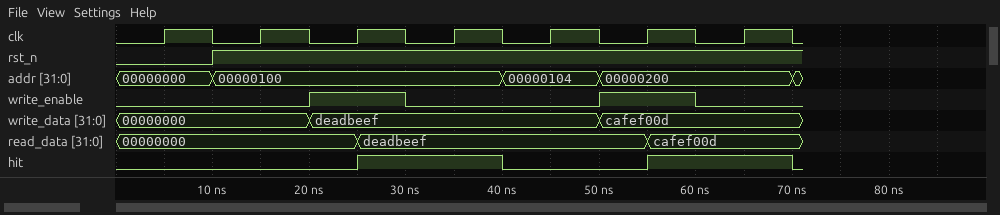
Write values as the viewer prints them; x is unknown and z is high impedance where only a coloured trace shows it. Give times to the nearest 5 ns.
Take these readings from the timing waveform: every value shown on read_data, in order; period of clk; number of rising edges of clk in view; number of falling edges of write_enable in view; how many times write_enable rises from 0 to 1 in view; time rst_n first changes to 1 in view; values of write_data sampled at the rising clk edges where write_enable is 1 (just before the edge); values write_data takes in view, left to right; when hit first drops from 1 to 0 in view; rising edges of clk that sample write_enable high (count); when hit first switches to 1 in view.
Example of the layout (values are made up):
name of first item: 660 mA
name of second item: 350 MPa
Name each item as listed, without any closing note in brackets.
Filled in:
every value shown on read_data, in order: 00000000, deadbeef, cafef00d
period of clk: 10 ns
number of rising edges of clk in view: 7
number of falling edges of write_enable in view: 2
how many times write_enable rises from 0 to 1 in view: 2
time rst_n first changes to 1 in view: 10 ns
values of write_data sampled at the rising clk edges where write_enable is 1: deadbeef, cafef00d
values write_data takes in view, left to right: 00000000, deadbeef, cafef00d
when hit first drops from 1 to 0 in view: 40 ns
rising edges of clk that sample write_enable high: 2
when hit first switches to 1 in view: 25 ns
